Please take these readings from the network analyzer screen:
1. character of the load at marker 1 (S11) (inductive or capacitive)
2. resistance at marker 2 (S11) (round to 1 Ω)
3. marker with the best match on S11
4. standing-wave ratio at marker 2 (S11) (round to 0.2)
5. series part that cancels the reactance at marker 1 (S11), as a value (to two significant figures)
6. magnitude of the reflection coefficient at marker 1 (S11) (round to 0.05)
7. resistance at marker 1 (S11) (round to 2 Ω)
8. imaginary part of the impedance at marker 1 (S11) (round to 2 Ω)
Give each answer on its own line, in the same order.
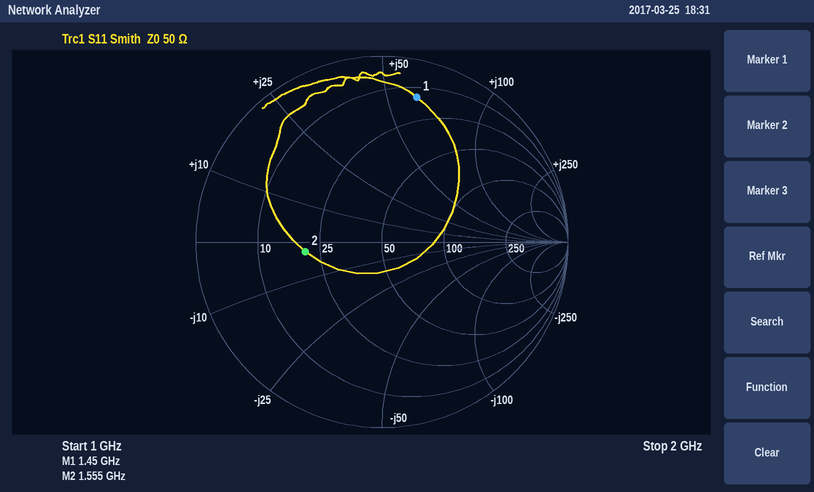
inductive
21 Ω
marker 2
2.4
1.8 pF
0.80
14 Ω
+62 Ω
